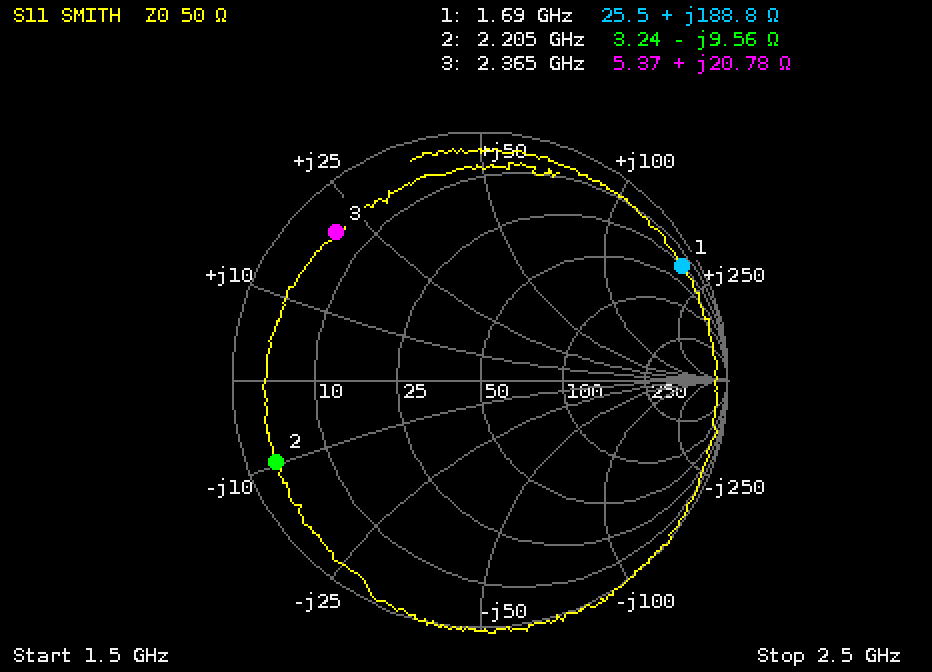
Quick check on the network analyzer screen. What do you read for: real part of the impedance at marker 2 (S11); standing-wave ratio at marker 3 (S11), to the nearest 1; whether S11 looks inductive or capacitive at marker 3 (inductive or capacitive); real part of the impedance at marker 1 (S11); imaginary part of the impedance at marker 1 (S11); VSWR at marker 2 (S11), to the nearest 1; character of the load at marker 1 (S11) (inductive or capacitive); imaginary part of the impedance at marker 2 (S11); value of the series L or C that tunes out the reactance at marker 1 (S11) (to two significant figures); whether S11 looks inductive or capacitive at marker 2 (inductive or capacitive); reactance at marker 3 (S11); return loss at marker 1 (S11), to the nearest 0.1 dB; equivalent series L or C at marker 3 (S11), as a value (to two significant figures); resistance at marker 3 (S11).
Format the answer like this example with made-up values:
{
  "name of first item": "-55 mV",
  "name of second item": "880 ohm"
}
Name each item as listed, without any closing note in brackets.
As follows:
{
  "real part of the impedance at marker 2": "3.24 Ω",
  "standing-wave ratio at marker 3 (S11), to the nearest 1": "11",
  "whether S11 looks inductive or capacitive at marker 3": "inductive",
  "real part of the impedance at marker 1": "25.5 Ω",
  "imaginary part of the impedance at marker 1": "+188.8 Ω",
  "VSWR at marker 2 (S11), to the nearest 1": "16",
  "character of the load at marker 1 (S11)": "inductive",
  "imaginary part of the impedance at marker 2": "-9.56 Ω",
  "value of the series L or C that tunes out the reactance at marker 1 (S11)": "500 fF",
  "whether S11 looks inductive or capacitive at marker 2": "capacitive",
  "reactance at marker 3": "+20.78 Ω",
  "return loss at marker 1 (S11), to the nearest 0.1 dB": "0.6 dB",
  "equivalent series L or C at marker 3 (S11), as a value": "1.4 nH",
  "resistance at marker 3": "5.37 Ω"
}
